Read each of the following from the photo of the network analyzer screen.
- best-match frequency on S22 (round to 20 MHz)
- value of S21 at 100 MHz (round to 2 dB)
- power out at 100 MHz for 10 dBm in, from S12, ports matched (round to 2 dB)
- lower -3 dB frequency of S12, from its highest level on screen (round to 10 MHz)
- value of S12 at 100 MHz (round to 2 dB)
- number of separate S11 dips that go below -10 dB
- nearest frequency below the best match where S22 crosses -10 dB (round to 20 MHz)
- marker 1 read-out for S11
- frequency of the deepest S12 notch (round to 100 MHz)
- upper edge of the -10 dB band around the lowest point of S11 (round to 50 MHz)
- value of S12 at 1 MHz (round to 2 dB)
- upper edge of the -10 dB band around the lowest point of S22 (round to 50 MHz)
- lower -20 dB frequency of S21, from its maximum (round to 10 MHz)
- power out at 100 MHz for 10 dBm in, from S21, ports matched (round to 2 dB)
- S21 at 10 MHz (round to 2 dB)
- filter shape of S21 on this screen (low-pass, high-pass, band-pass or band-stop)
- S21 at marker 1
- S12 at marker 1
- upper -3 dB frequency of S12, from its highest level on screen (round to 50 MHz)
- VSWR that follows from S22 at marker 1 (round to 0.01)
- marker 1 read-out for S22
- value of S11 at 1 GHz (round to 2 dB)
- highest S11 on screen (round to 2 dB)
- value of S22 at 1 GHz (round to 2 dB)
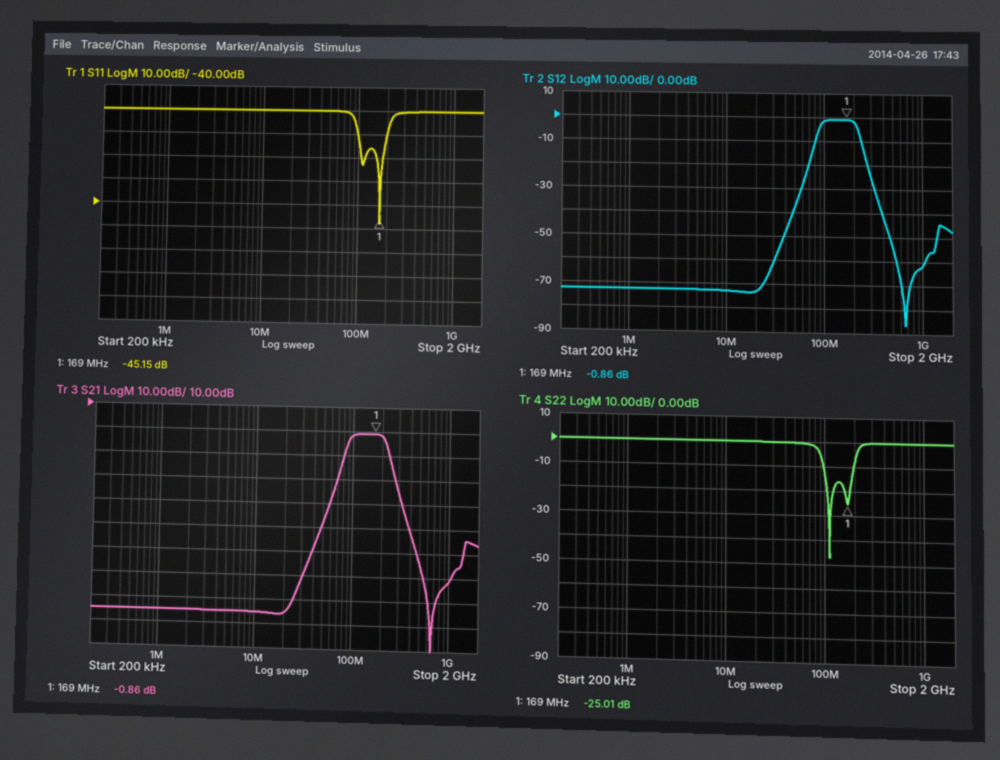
120 MHz
-2 dB
8 dBm
90 MHz
-2 dB
2
100 MHz
-45.15 dB
700 MHz
200 MHz
-72 dB
200 MHz
70 MHz
8 dBm
-76 dB
band-pass
-0.86 dB
-0.86 dB
200 MHz
1.12
-25.01 dB
0 dB
0 dB
0 dB
